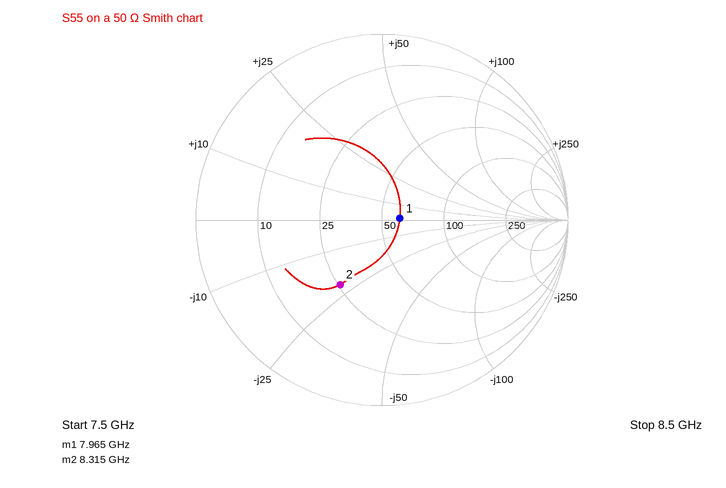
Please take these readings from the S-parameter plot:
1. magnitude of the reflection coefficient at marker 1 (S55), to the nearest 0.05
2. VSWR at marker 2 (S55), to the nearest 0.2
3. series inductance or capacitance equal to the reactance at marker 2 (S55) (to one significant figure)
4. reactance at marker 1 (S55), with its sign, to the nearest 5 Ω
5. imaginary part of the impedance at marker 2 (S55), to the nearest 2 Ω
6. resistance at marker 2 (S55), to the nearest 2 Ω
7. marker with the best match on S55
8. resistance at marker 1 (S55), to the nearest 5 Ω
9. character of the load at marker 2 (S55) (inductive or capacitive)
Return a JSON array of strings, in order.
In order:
["0.10", "2.4", "900 fF", "0 Ω", "-22 Ω", "26 Ω", "marker 1", "60 Ω", "capacitive"]
